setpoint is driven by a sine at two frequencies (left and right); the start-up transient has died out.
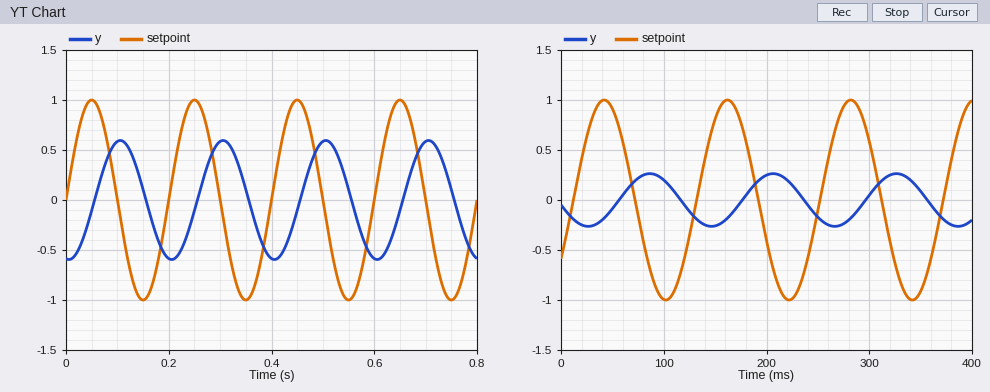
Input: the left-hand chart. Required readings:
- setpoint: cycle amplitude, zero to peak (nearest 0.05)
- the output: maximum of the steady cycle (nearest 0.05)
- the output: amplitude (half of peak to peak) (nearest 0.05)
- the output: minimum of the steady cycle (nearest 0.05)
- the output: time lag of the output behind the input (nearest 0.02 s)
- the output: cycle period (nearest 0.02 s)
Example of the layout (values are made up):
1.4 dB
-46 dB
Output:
1.00
0.60
0.60
-0.60
0.06 s
0.20 s
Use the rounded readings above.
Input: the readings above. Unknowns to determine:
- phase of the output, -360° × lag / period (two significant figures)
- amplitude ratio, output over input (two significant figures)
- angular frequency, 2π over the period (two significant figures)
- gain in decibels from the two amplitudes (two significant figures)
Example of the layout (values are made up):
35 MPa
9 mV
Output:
-110°
0.60
31 rad/s
-4.4 dB
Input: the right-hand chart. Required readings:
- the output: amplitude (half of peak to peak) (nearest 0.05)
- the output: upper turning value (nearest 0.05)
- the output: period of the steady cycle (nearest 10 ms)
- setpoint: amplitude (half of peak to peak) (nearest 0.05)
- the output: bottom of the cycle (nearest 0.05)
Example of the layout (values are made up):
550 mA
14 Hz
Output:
0.25
0.25
120 ms
1.00
-0.25
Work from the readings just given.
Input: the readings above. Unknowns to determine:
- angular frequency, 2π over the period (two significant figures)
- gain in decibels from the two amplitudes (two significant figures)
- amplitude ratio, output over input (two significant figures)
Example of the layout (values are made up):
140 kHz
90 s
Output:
0.052 rad/ms
-12 dB
0.25
